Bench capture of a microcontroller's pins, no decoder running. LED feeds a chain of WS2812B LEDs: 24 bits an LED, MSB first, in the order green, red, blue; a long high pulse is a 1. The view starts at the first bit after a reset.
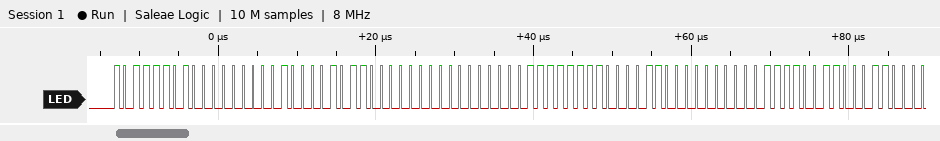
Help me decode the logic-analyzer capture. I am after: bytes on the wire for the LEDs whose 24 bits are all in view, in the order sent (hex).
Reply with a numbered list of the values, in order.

1. BD 00 42 C0 00 3F C3 00 3C
